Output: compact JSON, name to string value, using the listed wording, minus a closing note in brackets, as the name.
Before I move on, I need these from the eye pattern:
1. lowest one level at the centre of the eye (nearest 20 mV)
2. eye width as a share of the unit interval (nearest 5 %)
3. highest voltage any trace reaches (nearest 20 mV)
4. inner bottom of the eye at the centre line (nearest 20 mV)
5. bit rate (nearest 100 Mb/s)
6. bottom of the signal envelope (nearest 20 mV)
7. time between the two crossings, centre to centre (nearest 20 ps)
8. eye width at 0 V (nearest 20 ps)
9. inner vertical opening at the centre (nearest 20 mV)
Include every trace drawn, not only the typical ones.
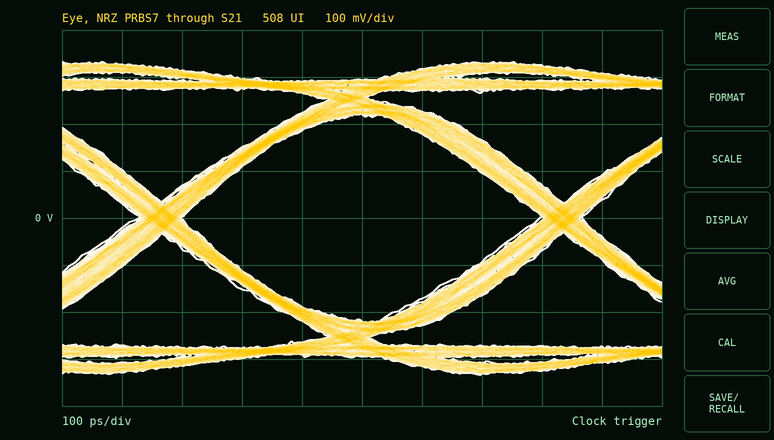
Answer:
{"lowest one level at the centre of the eye": "220 mV", "eye width as a share of the unit interval": "90 %", "highest voltage any trace reaches": "340 mV", "inner bottom of the eye at the centre line": "-220 mV", "bit rate": "1.5 Gb/s", "bottom of the signal envelope": "-340 mV", "time between the two crossings, centre to centre": "660 ps", "eye width at 0 V": "600 ps", "inner vertical opening at the centre": "440 mV"}
